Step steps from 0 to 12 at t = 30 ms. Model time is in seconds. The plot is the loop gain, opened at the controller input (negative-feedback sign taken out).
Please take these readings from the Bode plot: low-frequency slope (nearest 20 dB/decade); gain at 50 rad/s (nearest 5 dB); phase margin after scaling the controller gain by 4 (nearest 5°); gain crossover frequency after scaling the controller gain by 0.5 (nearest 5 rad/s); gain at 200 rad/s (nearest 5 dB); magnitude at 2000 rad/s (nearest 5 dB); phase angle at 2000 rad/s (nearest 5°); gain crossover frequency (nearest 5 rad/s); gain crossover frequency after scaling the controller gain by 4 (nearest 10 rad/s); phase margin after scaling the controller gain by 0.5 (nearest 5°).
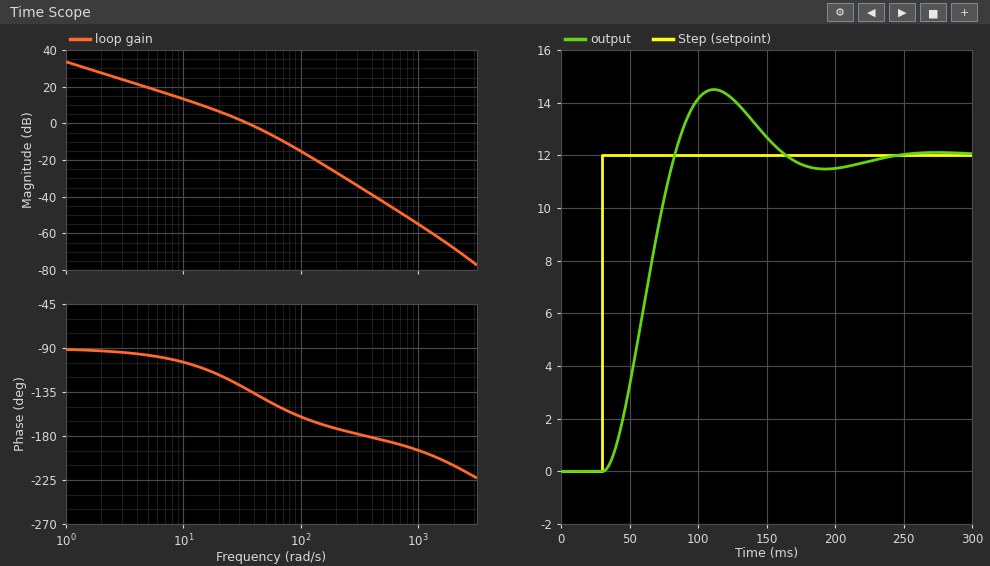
-20 dB/decade
-5 dB
25°
20 rad/s
-25 dB
-70 dB
-210°
35 rad/s
80 rad/s
60°
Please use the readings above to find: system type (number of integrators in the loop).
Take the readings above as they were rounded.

1
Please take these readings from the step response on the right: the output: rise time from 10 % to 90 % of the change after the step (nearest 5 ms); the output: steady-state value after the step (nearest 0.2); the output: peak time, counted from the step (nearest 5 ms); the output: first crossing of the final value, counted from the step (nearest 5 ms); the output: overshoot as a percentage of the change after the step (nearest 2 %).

35 ms
12.0
80 ms
55 ms
20 %
